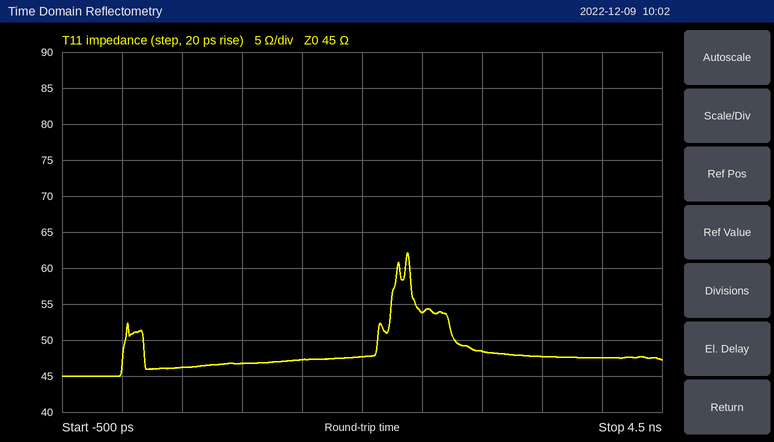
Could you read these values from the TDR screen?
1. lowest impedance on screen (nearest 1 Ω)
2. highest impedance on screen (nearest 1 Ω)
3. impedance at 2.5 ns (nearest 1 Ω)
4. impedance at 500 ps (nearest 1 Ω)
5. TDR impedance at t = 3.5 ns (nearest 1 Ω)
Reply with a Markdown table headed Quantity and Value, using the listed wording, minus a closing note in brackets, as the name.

| Quantity | Value |
|---|---|
| lowest impedance on screen | 45 Ω |
| highest impedance on screen | 62 Ω |
| impedance at 2.5 ns | 54 Ω |
| impedance at 500 ps | 46 Ω |
| TDR impedance at t = 3.5 ns | 48 Ω |
